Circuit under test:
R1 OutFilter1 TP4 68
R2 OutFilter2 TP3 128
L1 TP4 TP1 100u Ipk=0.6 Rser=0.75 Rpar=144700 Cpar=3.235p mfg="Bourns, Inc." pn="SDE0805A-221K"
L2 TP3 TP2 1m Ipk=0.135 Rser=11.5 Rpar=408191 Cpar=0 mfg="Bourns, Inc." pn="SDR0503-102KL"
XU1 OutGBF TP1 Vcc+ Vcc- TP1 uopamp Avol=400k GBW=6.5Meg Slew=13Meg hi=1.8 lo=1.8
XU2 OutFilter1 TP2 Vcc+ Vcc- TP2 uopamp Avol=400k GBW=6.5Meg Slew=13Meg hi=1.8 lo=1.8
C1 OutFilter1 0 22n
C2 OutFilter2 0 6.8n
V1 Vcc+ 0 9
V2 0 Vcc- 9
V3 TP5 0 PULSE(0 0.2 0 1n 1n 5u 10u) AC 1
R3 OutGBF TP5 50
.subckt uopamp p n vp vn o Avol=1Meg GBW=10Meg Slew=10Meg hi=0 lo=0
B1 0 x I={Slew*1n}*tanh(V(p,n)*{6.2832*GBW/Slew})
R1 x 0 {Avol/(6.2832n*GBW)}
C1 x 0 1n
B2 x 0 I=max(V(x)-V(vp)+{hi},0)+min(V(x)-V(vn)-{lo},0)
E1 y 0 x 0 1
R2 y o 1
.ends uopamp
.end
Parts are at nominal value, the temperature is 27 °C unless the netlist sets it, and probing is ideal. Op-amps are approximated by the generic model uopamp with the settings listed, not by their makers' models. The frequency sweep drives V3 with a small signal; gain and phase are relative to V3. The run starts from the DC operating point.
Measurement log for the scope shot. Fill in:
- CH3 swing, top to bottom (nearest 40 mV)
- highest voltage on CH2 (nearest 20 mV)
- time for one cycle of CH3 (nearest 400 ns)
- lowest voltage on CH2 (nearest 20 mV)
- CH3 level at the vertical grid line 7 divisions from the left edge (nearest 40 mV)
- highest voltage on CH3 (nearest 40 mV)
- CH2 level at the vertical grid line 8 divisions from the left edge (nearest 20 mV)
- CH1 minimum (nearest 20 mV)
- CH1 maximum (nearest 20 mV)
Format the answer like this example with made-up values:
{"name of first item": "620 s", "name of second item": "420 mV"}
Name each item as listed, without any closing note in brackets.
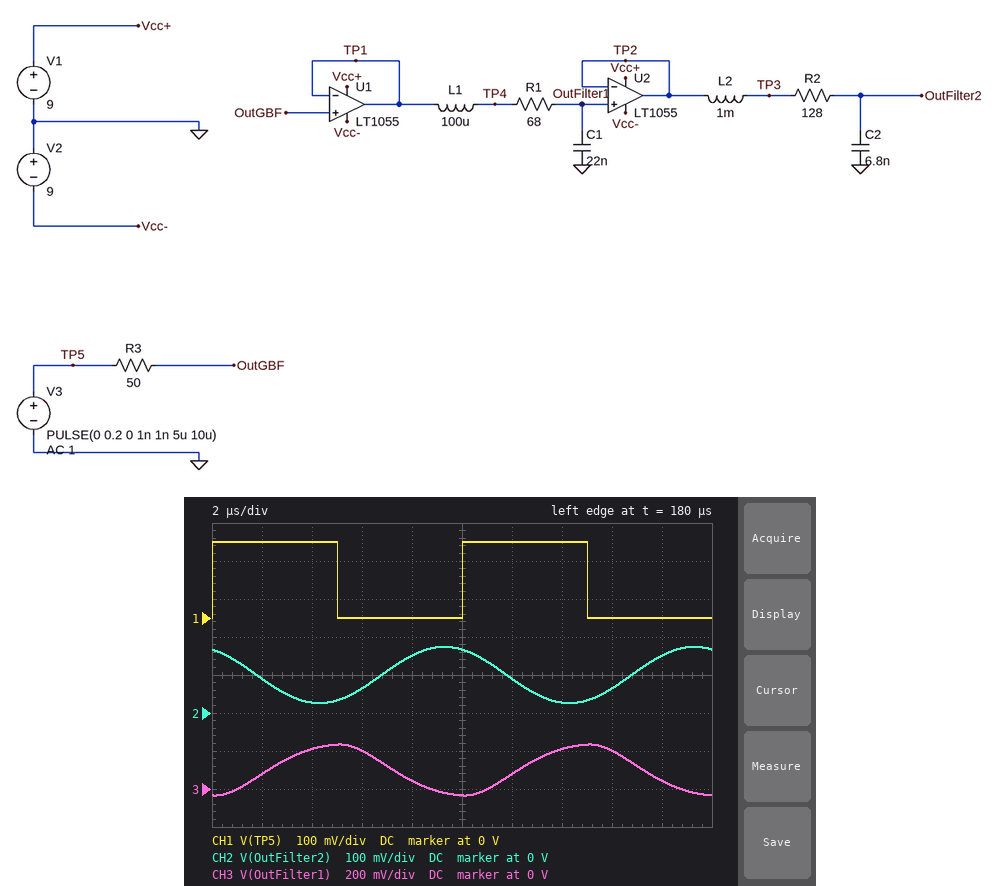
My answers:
{"CH3 swing, top to bottom": "280 mV", "highest voltage on CH2": "180 mV", "time for one cycle of CH3": "10.0 µs", "lowest voltage on CH2": "20 mV", "CH3 level at the vertical grid line 7 divisions from the left edge": "200 mV", "highest voltage on CH3": "240 mV", "CH2 level at the vertical grid line 8 divisions from the left edge": "60 mV", "CH1 minimum": "0 V", "CH1 maximum": "200 mV"}
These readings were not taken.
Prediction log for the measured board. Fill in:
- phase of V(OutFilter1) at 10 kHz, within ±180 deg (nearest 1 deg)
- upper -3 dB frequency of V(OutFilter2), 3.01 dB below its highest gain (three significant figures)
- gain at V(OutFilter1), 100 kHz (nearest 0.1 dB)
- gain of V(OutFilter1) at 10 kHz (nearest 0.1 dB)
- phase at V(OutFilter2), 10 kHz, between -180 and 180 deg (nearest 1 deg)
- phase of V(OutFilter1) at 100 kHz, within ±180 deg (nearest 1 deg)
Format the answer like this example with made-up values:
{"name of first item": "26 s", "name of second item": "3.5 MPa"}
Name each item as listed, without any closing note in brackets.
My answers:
{"phase of V(OutFilter1) at 10 kHz, within ±180 deg": "-6 deg", "upper -3 dB frequency of V(OutFilter2), 3.01 dB below its highest gain": "69.7 kHz", "gain at V(OutFilter1), 100 kHz": "0.4 dB", "gain of V(OutFilter1) at 10 kHz": "0 dB", "phase at V(OutFilter2), 10 kHz, between -180 and 180 deg": "-9 deg", "phase of V(OutFilter1) at 100 kHz, within ±180 deg": "-83 deg"}
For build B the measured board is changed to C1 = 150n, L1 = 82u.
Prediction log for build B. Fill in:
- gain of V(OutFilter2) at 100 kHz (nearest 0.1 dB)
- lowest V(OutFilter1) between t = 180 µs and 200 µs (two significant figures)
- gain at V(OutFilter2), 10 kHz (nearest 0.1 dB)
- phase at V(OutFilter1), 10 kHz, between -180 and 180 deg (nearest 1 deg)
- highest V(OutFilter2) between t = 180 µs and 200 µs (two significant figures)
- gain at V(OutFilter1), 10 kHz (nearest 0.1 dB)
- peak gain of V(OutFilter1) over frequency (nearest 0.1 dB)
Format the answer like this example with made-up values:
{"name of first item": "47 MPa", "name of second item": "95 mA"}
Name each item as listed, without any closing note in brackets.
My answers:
{"gain of V(OutFilter2) at 100 kHz": "-22.6 dB", "lowest V(OutFilter1) between t = 180 µs and 200 µs": "82 mV", "gain at V(OutFilter2), 10 kHz": "-1.0 dB", "phase at V(OutFilter1), 10 kHz, between -180 and 180 deg": "-34 deg", "highest V(OutFilter2) between t = 180 µs and 200 µs": "110 mV", "gain at V(OutFilter1), 10 kHz": "-1.2 dB", "peak gain of V(OutFilter1) over frequency": "0 dB"}
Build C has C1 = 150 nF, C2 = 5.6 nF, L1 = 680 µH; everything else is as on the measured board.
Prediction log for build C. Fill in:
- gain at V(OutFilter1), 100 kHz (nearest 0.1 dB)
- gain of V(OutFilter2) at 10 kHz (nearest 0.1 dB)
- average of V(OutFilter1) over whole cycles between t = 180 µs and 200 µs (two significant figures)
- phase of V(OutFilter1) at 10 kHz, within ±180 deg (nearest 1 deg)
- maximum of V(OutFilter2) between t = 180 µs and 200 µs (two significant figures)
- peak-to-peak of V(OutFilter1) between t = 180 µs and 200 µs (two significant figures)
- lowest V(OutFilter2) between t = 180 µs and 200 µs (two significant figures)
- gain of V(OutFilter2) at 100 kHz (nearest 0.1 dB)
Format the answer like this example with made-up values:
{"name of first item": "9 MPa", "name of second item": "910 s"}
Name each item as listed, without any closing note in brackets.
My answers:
{"gain at V(OutFilter1), 100 kHz": "-32.0 dB", "gain of V(OutFilter2) at 10 kHz": "1.3 dB", "average of V(OutFilter1) over whole cycles between t = 180 µs and 200 µs": "100 mV", "phase of V(OutFilter1) at 10 kHz, within ±180 deg": "-47 deg", "maximum of V(OutFilter2) between t = 180 µs and 200 µs": "100 mV", "peak-to-peak of V(OutFilter1) between t = 180 µs and 200 µs": "6.2 mV", "lowest V(OutFilter2) between t = 180 µs and 200 µs": "98 mV", "gain of V(OutFilter2) at 100 kHz": "-34.3 dB"}
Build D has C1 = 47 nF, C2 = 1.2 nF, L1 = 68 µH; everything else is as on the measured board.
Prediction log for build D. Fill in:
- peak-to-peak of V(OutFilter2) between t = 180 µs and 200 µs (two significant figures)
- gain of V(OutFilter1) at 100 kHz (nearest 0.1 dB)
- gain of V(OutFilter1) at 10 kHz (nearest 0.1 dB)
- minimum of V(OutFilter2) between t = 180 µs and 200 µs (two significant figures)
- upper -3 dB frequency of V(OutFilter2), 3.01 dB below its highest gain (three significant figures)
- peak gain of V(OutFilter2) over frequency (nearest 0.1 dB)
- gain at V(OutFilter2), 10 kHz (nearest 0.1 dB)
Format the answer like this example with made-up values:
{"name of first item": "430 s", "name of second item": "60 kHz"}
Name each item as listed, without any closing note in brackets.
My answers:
{"peak-to-peak of V(OutFilter2) between t = 180 µs and 200 µs": "230 mV", "gain of V(OutFilter1) at 100 kHz": "-6.2 dB", "gain of V(OutFilter1) at 10 kHz": "-0.1 dB", "minimum of V(OutFilter2) between t = 180 µs and 200 µs": "-15 mV", "upper -3 dB frequency of V(OutFilter2), 3.01 dB below its highest gain": "153 kHz", "peak gain of V(OutFilter2) over frequency": "5.8 dB", "gain at V(OutFilter2), 10 kHz": "0 dB"}
